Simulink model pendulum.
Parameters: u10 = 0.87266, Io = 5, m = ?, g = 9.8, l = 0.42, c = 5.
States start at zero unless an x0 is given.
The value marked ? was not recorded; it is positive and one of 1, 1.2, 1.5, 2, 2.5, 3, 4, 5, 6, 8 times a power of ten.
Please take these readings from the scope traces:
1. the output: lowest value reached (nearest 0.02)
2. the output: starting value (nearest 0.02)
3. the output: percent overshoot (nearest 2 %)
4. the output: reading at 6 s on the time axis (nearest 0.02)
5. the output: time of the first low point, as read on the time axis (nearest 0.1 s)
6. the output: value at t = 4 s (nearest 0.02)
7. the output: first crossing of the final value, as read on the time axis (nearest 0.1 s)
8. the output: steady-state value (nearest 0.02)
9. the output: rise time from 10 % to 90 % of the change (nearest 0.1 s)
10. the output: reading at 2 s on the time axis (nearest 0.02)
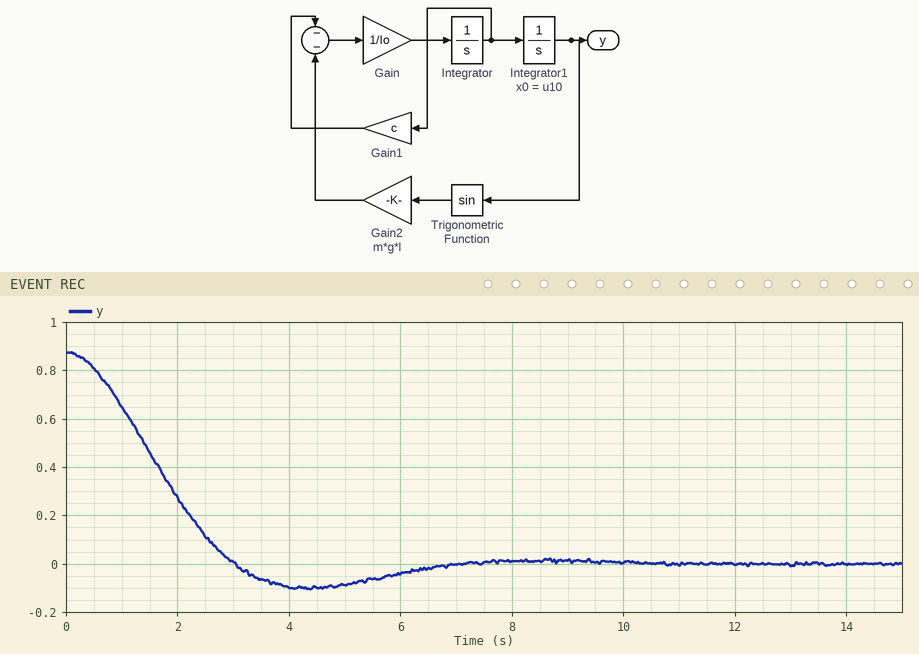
-0.10
0.88
12 %
-0.04
4.3 s
-0.10
3.0 s
0.00
2.0 s
0.28
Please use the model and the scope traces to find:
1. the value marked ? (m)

1
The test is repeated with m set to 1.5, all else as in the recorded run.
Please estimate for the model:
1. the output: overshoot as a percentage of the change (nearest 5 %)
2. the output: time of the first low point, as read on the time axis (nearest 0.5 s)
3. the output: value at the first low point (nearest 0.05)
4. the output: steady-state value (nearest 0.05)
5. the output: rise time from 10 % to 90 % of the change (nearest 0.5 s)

20 %
3.5 s
-0.15
0.00
1.5 s
